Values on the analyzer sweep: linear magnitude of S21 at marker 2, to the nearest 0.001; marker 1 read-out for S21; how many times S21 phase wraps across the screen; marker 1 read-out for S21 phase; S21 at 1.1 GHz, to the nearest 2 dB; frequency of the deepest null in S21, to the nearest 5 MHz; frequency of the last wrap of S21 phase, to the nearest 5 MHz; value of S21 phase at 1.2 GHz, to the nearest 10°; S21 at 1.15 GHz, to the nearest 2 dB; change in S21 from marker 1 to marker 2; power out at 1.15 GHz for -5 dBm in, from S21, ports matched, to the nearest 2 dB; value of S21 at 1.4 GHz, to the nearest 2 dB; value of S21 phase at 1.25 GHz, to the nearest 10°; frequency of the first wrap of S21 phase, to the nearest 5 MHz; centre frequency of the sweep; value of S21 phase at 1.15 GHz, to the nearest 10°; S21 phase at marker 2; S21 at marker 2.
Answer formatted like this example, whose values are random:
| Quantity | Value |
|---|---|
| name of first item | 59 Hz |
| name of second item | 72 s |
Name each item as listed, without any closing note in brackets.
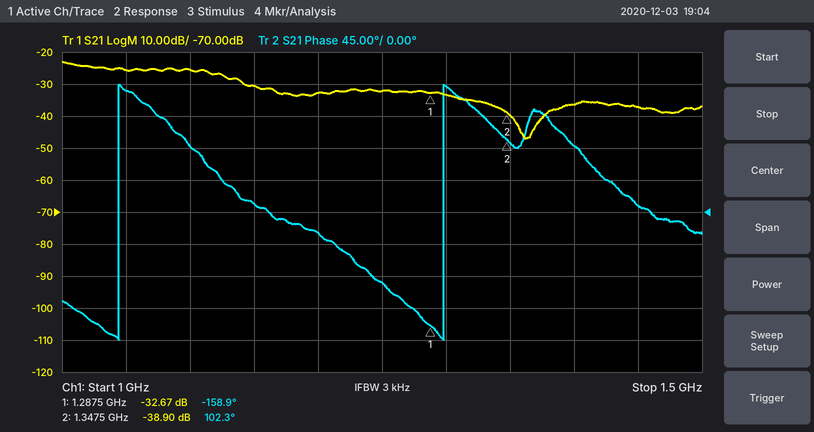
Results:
| Quantity | Value |
|---|---|
| linear magnitude of S21 at marker 2, to the nearest 0.001 | 0.011 |
| marker 1 read-out for S21 | -32.67 dB |
| how many times S21 phase wraps across the screen | 2 |
| marker 1 read-out for S21 phase | -158.9° |
| S21 at 1.1 GHz, to the nearest 2 dB | -26 dB |
| frequency of the deepest null in S21, to the nearest 5 MHz | 1.360 GHz |
| frequency of the last wrap of S21 phase, to the nearest 5 MHz | 1.300 GHz |
| value of S21 phase at 1.2 GHz, to the nearest 10° | -30° |
| S21 at 1.15 GHz, to the nearest 2 dB | -30 dB |
| change in S21 from marker 1 to marker 2 | -6.23 dB |
| power out at 1.15 GHz for -5 dBm in, from S21, ports matched, to the nearest 2 dB | -36 dBm |
| value of S21 at 1.4 GHz, to the nearest 2 dB | -36 dB |
| value of S21 phase at 1.25 GHz, to the nearest 10° | -100° |
| frequency of the first wrap of S21 phase, to the nearest 5 MHz | 1.045 GHz |
| centre frequency of the sweep | 1.25 GHz |
| value of S21 phase at 1.15 GHz, to the nearest 10° | 10° |
| S21 phase at marker 2 | 102.3° |
| S21 at marker 2 | -38.90 dB |
